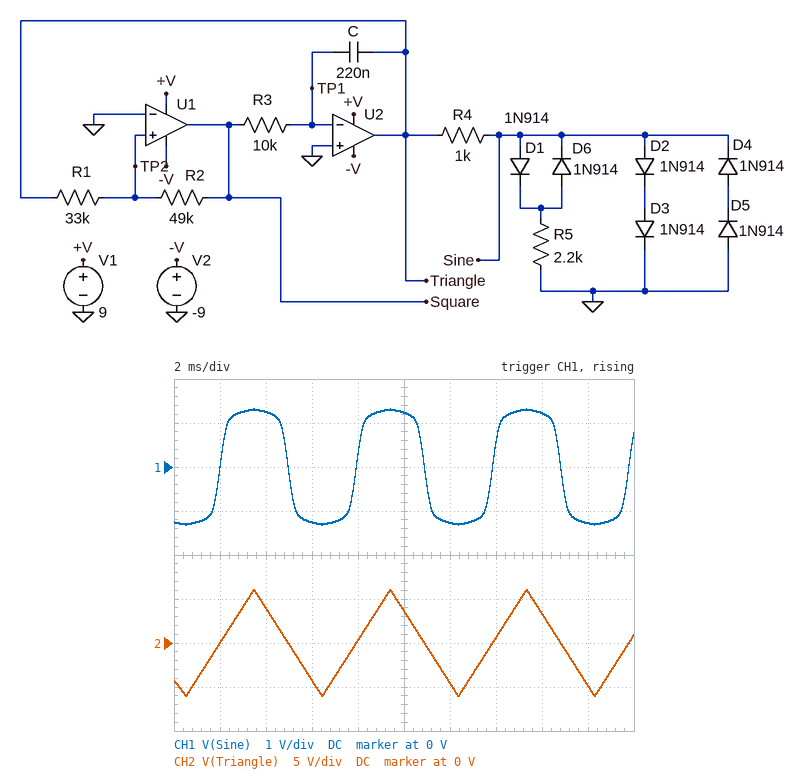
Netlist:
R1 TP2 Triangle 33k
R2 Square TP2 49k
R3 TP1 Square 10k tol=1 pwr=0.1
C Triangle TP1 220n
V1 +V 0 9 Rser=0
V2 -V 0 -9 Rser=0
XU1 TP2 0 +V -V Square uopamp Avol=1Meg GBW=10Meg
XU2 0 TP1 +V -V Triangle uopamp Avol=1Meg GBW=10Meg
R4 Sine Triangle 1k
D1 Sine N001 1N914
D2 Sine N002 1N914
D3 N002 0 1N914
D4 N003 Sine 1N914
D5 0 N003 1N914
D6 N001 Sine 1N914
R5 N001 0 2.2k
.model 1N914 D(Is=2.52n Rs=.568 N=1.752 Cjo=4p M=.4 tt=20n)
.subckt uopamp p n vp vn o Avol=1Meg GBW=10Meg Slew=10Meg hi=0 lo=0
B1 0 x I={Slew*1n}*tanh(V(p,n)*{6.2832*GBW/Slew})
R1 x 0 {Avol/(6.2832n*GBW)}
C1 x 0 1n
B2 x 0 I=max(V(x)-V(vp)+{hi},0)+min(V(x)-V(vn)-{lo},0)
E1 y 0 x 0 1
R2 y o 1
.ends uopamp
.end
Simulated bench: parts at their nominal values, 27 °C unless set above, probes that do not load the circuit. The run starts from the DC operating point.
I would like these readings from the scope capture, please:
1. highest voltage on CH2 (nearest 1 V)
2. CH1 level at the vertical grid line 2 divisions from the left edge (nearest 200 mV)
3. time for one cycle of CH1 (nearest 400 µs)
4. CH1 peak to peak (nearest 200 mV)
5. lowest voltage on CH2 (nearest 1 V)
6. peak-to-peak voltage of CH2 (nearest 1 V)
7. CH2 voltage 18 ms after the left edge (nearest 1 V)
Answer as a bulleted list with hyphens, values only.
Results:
- 6 V
- 1.2 V
- 6.0 ms
- 2.6 V
- -6 V
- 12 V
- -5 V
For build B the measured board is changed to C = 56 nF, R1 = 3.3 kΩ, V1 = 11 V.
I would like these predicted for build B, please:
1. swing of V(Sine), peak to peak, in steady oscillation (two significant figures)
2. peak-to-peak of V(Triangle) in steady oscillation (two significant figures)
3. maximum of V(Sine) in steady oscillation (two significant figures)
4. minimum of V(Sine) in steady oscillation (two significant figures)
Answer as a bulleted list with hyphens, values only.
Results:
- 1.2 V
- 1.4 V
- 570 mV
- -670 mV
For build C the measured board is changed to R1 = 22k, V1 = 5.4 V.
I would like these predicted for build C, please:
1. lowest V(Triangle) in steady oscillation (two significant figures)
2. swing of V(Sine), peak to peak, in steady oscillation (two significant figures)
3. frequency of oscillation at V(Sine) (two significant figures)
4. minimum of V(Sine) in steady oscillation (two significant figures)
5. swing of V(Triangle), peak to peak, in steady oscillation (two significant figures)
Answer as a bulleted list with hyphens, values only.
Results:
- -2.4 V
- 2.4 V
- 240 Hz
- -1.2 V
- 6.5 V
